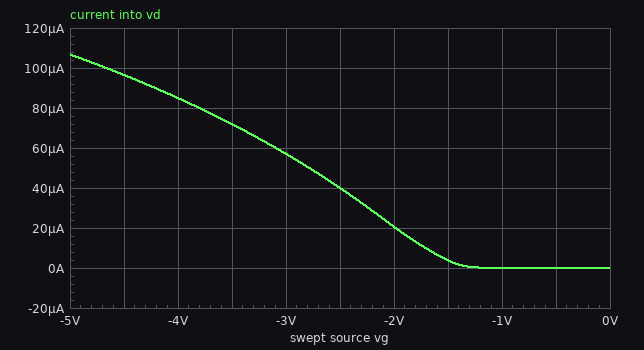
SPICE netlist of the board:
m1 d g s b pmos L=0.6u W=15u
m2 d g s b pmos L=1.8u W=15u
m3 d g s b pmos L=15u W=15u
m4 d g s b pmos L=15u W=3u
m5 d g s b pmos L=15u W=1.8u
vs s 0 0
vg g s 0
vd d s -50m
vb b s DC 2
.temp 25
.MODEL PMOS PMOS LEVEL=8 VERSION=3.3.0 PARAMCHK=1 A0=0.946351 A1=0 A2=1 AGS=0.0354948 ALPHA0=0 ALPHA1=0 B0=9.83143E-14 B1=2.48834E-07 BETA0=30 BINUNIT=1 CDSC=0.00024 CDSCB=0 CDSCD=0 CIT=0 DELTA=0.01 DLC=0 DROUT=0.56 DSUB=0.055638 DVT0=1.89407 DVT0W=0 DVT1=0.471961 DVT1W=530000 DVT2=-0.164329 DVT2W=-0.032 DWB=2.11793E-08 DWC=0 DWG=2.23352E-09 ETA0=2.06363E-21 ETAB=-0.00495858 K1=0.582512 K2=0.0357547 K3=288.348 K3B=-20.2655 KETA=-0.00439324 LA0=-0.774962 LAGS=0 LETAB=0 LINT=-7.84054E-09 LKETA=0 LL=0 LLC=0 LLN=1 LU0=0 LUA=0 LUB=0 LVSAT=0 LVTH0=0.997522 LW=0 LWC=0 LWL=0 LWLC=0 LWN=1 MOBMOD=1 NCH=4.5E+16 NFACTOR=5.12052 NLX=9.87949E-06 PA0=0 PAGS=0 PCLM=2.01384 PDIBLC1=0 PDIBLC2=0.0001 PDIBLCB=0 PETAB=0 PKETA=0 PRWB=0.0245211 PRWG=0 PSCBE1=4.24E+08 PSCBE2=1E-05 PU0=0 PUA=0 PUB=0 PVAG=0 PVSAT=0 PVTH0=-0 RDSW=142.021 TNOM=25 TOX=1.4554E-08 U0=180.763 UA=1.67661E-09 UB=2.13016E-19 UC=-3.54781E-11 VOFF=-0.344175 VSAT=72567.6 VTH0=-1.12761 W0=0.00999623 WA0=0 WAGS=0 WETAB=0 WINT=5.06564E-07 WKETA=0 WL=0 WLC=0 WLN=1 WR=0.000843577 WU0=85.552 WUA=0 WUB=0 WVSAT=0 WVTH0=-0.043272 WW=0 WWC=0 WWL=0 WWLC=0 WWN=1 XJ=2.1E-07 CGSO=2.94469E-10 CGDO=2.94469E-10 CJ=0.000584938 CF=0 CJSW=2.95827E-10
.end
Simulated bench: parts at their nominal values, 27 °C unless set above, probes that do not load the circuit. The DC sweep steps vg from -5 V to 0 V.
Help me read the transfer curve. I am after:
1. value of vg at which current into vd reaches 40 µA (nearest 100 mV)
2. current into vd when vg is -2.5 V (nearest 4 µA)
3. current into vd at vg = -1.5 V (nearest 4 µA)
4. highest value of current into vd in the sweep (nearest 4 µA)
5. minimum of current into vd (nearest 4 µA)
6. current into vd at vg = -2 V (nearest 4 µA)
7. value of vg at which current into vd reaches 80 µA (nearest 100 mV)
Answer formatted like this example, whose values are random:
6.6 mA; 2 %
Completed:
-2.5 V; 40 µA; 4 µA; 108 µA; 0 A; 20 µA; -3.8 V
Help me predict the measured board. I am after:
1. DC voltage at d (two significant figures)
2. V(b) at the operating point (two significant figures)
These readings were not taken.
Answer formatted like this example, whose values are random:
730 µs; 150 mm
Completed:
-50 mV; 2.0 V
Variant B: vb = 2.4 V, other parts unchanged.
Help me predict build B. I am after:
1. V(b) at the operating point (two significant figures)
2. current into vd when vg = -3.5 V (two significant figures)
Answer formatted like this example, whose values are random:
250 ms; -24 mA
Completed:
2.4 V; 69 µA
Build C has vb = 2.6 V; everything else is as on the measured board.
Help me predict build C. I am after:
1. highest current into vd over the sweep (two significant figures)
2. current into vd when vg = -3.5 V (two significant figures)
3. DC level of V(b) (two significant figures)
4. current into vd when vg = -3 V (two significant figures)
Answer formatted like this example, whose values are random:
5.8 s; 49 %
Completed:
100 µA; 68 µA; 2.6 V; 53 µA
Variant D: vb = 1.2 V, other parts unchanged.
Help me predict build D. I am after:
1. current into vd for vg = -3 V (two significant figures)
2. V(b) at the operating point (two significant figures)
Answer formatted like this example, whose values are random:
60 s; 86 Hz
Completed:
63 µA; 1.2 V
